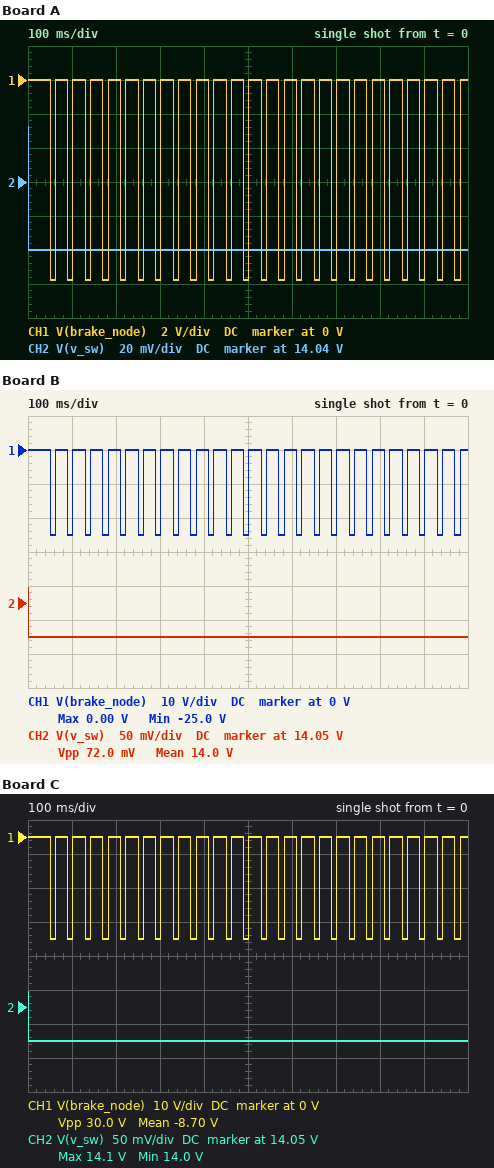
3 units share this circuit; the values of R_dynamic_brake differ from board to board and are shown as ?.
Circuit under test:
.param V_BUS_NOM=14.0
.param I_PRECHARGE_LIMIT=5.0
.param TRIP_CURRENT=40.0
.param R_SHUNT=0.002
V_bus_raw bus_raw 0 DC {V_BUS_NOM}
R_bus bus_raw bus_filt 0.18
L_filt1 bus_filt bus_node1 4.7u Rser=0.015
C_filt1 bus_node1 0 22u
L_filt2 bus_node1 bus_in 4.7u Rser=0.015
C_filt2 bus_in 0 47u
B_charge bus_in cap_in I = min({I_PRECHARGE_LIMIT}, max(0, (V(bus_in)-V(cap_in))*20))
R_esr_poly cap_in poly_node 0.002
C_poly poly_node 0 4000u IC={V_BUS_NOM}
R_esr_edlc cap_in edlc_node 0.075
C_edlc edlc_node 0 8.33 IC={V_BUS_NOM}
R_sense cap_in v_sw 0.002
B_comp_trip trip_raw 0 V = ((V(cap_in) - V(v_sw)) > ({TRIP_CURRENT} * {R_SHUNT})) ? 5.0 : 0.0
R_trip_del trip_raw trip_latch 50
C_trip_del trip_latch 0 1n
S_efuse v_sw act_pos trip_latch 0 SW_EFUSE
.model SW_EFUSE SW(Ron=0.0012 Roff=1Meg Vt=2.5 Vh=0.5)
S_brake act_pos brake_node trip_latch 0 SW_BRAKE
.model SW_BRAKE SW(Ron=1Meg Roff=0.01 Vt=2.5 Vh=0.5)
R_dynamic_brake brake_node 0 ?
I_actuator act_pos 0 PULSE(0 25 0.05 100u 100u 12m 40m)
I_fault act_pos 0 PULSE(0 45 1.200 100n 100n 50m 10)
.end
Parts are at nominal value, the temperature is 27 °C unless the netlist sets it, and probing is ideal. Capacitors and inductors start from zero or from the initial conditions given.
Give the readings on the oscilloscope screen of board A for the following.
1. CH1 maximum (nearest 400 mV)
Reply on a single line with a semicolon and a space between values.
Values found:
0 V
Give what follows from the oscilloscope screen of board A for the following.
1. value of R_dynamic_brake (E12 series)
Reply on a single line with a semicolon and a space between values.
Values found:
0.47 Ω
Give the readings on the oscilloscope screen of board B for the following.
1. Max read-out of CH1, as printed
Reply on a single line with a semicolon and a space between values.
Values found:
0.00 V
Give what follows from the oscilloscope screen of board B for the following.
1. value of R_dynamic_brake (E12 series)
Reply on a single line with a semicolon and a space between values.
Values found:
1 Ω
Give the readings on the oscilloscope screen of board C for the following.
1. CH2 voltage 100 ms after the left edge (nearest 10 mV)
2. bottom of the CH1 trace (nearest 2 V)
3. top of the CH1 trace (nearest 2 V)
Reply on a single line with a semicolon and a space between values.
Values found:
14.00 V; -30 V; 0 V
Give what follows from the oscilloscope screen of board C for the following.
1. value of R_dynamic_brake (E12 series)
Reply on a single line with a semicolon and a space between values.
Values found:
1.2 Ω
